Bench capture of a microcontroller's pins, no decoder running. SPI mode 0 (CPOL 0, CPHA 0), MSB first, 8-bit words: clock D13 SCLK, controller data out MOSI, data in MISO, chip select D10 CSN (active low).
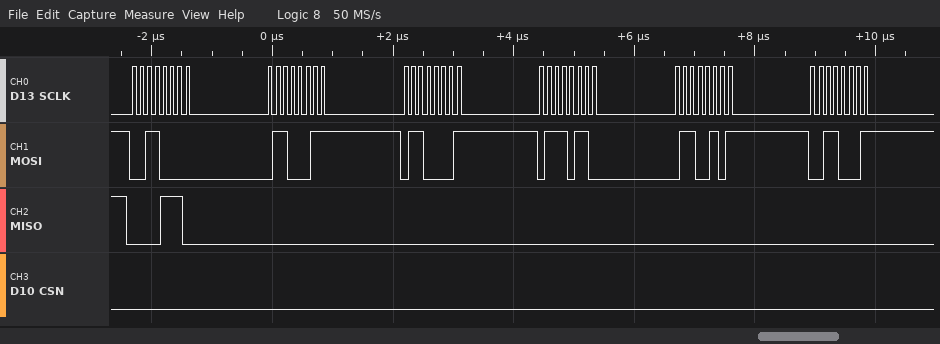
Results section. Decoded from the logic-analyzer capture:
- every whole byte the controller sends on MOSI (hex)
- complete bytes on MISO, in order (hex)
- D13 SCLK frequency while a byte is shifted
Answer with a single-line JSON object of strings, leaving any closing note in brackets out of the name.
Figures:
{"every whole byte the controller sends on MOSI": "30 63 61 76 65 31", "complete bytes on MISO, in order": "0E 00 00 00 00 00", "D13 SCLK frequency while a byte is shifted": "8 MHz"}
